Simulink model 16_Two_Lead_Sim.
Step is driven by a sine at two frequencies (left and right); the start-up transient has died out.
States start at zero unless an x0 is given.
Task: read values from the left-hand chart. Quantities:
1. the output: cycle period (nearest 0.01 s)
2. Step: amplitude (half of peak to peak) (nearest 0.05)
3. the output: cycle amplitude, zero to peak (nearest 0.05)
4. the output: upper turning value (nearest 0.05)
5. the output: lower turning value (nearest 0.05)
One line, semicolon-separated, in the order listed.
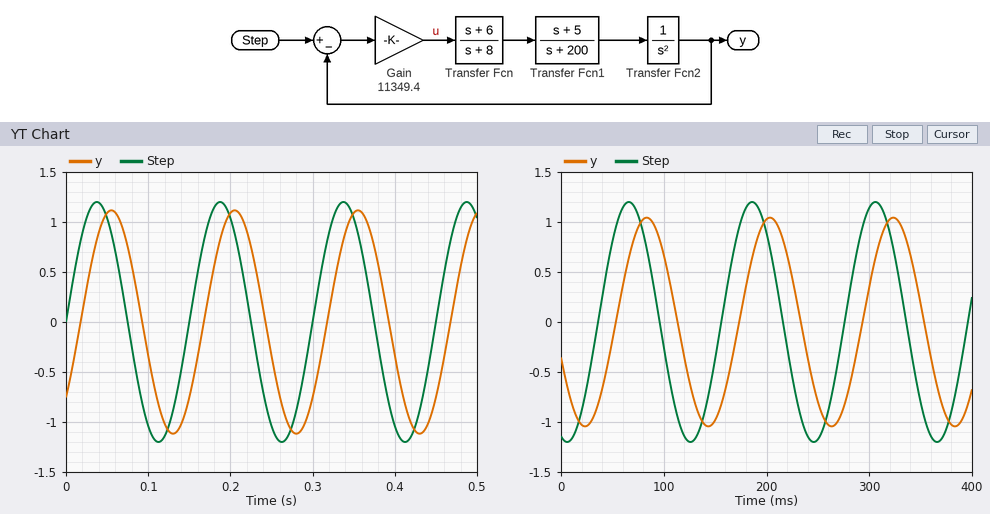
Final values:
0.15 s; 1.20; 1.10; 1.10; -1.10
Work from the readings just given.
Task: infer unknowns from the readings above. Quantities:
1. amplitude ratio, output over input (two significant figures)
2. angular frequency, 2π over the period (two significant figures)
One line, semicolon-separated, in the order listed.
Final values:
0.92; 42 rad/s
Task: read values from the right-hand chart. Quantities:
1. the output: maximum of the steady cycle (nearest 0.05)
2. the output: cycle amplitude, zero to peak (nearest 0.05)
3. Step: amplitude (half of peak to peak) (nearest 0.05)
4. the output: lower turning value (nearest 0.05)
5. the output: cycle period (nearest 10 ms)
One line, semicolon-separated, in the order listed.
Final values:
1.05; 1.05; 1.20; -1.05; 120 ms
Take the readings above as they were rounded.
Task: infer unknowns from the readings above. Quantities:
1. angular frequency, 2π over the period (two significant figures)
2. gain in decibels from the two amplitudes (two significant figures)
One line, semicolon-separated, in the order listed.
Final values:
0.052 rad/ms; -1.2 dB
